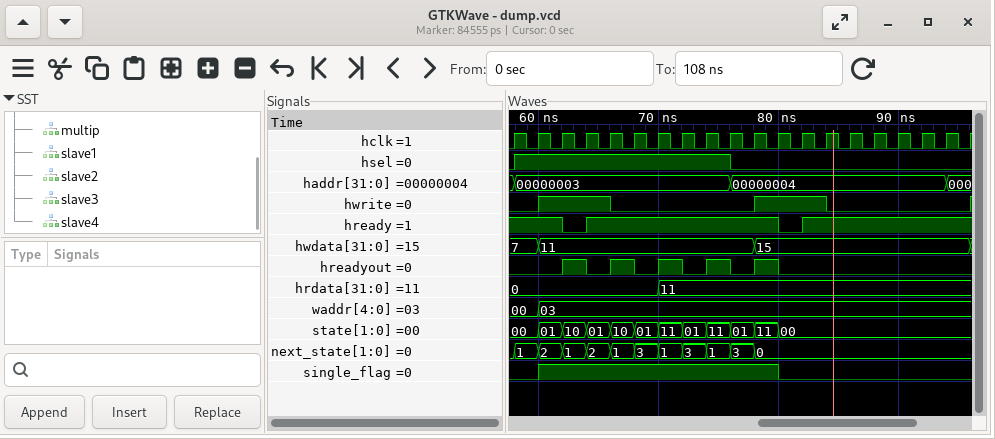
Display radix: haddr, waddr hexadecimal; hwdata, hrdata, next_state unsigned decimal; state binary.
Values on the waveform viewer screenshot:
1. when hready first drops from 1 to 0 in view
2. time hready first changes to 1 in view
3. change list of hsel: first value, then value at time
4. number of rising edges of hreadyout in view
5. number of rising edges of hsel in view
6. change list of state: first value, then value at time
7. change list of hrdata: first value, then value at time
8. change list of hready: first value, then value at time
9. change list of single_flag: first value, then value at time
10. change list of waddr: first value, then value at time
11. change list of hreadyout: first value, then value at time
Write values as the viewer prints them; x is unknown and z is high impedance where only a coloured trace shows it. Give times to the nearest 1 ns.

62 ns
64 ns
0, 1 at 58 ns, 0 at 76 ns
5
1
00, 01 at 60 ns, 10 at 62 ns, 01 at 64 ns, 10 at 66 ns, 01 at 68 ns, 11 at 70 ns, 01 at 72 ns, 11 at 74 ns, 01 at 76 ns, 11 at 78 ns, 00 at 80 ns
0, 11 at 70 ns
1, 0 at 62 ns, 1 at 64 ns, 0 at 80 ns, 1 at 82 ns
0, 1 at 60 ns, 0 at 80 ns
00, 03 at 60 ns
0, 1 at 62 ns, 0 at 64 ns, 1 at 66 ns, 0 at 68 ns, 1 at 70 ns, 0 at 72 ns, 1 at 74 ns, 0 at 76 ns, 1 at 78 ns, 0 at 80 ns
